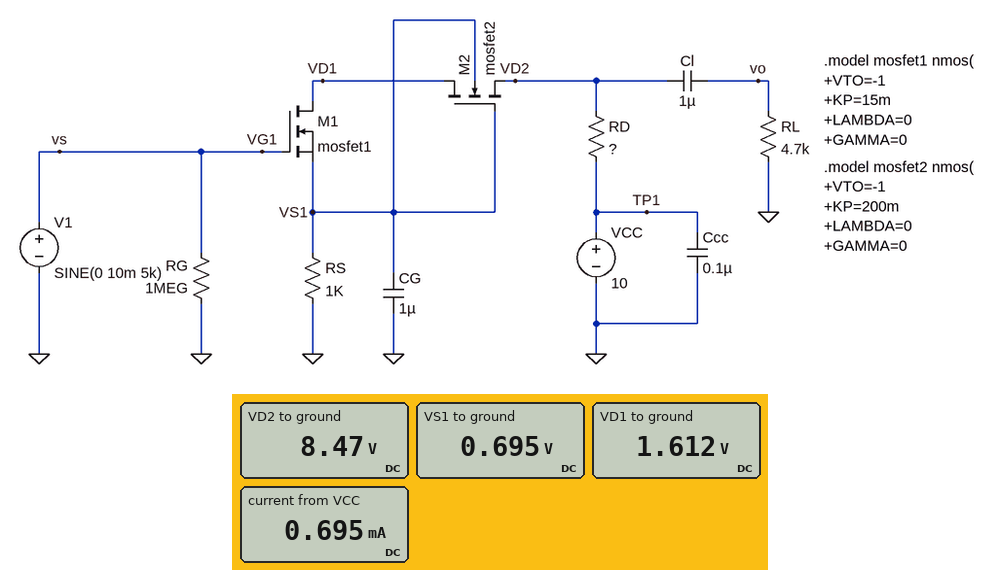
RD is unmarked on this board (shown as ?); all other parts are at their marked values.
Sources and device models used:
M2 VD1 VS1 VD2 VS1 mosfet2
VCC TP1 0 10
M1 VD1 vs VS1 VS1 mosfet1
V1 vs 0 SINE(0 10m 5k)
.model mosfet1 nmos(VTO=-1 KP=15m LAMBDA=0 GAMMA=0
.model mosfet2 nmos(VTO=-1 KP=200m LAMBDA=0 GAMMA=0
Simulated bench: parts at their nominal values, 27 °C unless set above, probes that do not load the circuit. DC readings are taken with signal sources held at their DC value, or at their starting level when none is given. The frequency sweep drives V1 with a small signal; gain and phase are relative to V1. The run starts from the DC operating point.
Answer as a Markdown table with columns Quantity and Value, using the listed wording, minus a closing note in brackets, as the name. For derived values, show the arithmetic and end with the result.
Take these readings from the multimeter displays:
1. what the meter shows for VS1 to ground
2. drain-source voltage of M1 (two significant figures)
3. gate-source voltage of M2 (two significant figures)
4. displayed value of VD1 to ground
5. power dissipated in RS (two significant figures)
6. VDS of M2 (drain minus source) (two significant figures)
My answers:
| Quantity | Value |
|---|---|
| what the meter shows for VS1 to ground | 0.695 V |
| drain-source voltage of M1 | 1.612 V - 695 mV = 920 mV |
| gate-source voltage of M2 | 695 mV - 8.47 V = -7.8 V |
| displayed value of VD1 to ground | 1.612 V |
| power dissipated in RS | (695 mV)^2 / 1 kΩ = 480 µW |
| VDS of M2 (drain minus source) | 1.612 V - 8.47 V = -6.9 V |
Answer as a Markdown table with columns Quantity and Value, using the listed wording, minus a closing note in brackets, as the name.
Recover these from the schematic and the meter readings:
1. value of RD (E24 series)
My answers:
| Quantity | Value |
|---|---|
| value of RD | 2.2 kΩ |
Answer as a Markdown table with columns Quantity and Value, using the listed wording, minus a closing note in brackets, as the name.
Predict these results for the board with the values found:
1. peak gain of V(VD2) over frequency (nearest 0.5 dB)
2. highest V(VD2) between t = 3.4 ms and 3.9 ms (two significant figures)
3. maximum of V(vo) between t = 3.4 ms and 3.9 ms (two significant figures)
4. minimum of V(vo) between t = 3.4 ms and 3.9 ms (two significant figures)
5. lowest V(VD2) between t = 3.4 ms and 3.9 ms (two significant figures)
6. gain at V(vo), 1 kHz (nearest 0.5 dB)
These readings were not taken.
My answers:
| Quantity | Value |
|---|---|
| peak gain of V(VD2) over frequency | 16.5 dB |
| highest V(VD2) between t = 3.4 ms and 3.9 ms | 8.5 V |
| maximum of V(vo) between t = 3.4 ms and 3.9 ms | 67 mV |
| minimum of V(vo) between t = 3.4 ms and 3.9 ms | -68 mV |
| lowest V(VD2) between t = 3.4 ms and 3.9 ms | 8.4 V |
| gain at V(vo), 1 kHz | 14.5 dB |
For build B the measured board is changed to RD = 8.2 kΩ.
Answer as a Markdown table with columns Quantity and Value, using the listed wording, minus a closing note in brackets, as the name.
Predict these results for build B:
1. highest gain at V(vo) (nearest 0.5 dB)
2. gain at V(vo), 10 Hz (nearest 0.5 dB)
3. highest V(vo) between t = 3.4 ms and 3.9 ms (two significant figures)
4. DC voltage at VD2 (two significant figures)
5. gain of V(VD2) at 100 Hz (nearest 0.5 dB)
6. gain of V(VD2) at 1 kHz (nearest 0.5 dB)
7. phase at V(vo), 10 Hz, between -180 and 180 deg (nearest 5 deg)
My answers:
| Quantity | Value |
|---|---|
| highest gain at V(vo) | 22.5 dB |
| gain at V(vo), 10 Hz | 4.0 dB |
| highest V(vo) between t = 3.4 ms and 3.9 ms | 130 mV |
| DC voltage at VD2 | 4.3 V |
| gain of V(VD2) at 100 Hz | 9.5 dB |
| gain of V(VD2) at 1 kHz | 20.5 dB |
| phase at V(vo), 10 Hz, between -180 and 180 deg | -125 deg |
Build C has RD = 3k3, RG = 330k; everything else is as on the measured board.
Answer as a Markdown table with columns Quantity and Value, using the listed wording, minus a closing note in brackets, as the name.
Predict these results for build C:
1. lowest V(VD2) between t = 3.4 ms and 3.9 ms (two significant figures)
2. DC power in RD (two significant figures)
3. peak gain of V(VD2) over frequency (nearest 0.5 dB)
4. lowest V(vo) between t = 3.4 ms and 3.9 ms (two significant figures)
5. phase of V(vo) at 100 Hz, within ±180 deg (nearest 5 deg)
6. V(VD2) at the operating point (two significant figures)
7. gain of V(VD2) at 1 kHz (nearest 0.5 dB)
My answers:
| Quantity | Value |
|---|---|
| lowest V(VD2) between t = 3.4 ms and 3.9 ms | 7.6 V |
| DC power in RD | 1.6 mW |
| peak gain of V(VD2) over frequency | 19.0 dB |
| lowest V(vo) between t = 3.4 ms and 3.9 ms | -88 mV |
| phase of V(vo) at 100 Hz, within ±180 deg | -145 deg |
| V(VD2) at the operating point | 7.7 V |
| gain of V(VD2) at 1 kHz | 16.5 dB |
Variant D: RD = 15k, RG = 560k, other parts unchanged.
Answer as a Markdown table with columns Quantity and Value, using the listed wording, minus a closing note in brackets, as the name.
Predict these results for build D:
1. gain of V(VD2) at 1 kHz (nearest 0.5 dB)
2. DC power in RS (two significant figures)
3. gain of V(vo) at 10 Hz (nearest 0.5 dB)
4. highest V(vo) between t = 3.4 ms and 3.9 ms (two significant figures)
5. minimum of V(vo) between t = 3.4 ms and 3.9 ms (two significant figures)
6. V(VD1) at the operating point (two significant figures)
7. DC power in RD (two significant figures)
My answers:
| Quantity | Value |
|---|---|
| gain of V(VD2) at 1 kHz | -6.5 dB |
| DC power in RS | 380 µW |
| gain of V(vo) at 10 Hz | -18.0 dB |
| highest V(vo) between t = 3.4 ms and 3.9 ms | 4.9 mV |
| minimum of V(vo) between t = 3.4 ms and 3.9 ms | -4.6 mV |
| V(VD1) at the operating point | 750 mV |
| DC power in RD | 5.7 mW |
